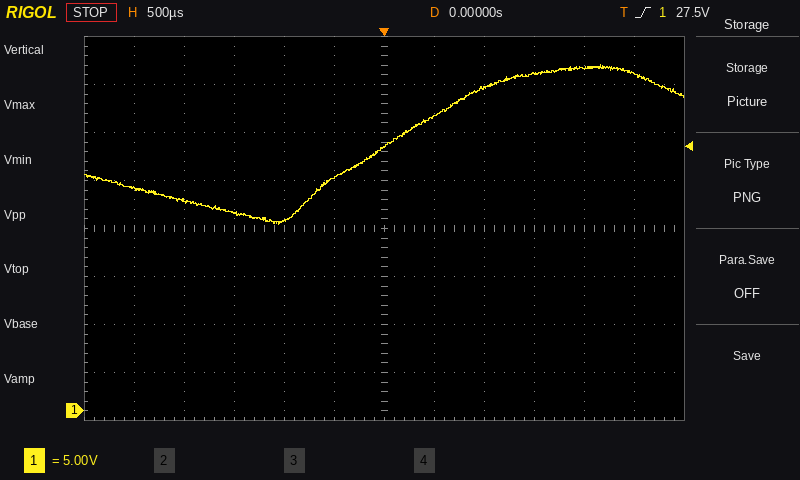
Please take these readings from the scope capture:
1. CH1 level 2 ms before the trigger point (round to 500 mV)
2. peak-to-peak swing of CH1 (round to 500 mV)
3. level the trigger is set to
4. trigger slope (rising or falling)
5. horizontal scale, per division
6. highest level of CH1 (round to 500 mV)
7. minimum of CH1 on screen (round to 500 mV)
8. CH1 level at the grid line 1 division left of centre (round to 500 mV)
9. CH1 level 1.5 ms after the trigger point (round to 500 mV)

22.0 V
16.5 V
27.5 V
rising
500 µs
36.0 V
19.5 V
24.5 V
35.0 V
